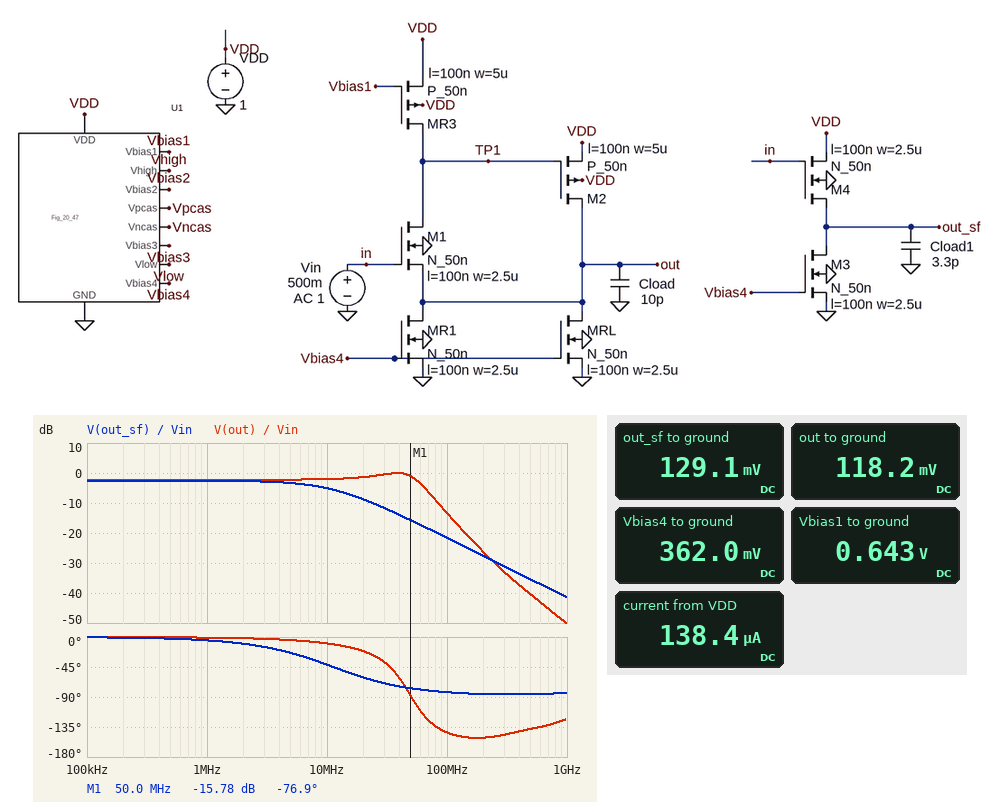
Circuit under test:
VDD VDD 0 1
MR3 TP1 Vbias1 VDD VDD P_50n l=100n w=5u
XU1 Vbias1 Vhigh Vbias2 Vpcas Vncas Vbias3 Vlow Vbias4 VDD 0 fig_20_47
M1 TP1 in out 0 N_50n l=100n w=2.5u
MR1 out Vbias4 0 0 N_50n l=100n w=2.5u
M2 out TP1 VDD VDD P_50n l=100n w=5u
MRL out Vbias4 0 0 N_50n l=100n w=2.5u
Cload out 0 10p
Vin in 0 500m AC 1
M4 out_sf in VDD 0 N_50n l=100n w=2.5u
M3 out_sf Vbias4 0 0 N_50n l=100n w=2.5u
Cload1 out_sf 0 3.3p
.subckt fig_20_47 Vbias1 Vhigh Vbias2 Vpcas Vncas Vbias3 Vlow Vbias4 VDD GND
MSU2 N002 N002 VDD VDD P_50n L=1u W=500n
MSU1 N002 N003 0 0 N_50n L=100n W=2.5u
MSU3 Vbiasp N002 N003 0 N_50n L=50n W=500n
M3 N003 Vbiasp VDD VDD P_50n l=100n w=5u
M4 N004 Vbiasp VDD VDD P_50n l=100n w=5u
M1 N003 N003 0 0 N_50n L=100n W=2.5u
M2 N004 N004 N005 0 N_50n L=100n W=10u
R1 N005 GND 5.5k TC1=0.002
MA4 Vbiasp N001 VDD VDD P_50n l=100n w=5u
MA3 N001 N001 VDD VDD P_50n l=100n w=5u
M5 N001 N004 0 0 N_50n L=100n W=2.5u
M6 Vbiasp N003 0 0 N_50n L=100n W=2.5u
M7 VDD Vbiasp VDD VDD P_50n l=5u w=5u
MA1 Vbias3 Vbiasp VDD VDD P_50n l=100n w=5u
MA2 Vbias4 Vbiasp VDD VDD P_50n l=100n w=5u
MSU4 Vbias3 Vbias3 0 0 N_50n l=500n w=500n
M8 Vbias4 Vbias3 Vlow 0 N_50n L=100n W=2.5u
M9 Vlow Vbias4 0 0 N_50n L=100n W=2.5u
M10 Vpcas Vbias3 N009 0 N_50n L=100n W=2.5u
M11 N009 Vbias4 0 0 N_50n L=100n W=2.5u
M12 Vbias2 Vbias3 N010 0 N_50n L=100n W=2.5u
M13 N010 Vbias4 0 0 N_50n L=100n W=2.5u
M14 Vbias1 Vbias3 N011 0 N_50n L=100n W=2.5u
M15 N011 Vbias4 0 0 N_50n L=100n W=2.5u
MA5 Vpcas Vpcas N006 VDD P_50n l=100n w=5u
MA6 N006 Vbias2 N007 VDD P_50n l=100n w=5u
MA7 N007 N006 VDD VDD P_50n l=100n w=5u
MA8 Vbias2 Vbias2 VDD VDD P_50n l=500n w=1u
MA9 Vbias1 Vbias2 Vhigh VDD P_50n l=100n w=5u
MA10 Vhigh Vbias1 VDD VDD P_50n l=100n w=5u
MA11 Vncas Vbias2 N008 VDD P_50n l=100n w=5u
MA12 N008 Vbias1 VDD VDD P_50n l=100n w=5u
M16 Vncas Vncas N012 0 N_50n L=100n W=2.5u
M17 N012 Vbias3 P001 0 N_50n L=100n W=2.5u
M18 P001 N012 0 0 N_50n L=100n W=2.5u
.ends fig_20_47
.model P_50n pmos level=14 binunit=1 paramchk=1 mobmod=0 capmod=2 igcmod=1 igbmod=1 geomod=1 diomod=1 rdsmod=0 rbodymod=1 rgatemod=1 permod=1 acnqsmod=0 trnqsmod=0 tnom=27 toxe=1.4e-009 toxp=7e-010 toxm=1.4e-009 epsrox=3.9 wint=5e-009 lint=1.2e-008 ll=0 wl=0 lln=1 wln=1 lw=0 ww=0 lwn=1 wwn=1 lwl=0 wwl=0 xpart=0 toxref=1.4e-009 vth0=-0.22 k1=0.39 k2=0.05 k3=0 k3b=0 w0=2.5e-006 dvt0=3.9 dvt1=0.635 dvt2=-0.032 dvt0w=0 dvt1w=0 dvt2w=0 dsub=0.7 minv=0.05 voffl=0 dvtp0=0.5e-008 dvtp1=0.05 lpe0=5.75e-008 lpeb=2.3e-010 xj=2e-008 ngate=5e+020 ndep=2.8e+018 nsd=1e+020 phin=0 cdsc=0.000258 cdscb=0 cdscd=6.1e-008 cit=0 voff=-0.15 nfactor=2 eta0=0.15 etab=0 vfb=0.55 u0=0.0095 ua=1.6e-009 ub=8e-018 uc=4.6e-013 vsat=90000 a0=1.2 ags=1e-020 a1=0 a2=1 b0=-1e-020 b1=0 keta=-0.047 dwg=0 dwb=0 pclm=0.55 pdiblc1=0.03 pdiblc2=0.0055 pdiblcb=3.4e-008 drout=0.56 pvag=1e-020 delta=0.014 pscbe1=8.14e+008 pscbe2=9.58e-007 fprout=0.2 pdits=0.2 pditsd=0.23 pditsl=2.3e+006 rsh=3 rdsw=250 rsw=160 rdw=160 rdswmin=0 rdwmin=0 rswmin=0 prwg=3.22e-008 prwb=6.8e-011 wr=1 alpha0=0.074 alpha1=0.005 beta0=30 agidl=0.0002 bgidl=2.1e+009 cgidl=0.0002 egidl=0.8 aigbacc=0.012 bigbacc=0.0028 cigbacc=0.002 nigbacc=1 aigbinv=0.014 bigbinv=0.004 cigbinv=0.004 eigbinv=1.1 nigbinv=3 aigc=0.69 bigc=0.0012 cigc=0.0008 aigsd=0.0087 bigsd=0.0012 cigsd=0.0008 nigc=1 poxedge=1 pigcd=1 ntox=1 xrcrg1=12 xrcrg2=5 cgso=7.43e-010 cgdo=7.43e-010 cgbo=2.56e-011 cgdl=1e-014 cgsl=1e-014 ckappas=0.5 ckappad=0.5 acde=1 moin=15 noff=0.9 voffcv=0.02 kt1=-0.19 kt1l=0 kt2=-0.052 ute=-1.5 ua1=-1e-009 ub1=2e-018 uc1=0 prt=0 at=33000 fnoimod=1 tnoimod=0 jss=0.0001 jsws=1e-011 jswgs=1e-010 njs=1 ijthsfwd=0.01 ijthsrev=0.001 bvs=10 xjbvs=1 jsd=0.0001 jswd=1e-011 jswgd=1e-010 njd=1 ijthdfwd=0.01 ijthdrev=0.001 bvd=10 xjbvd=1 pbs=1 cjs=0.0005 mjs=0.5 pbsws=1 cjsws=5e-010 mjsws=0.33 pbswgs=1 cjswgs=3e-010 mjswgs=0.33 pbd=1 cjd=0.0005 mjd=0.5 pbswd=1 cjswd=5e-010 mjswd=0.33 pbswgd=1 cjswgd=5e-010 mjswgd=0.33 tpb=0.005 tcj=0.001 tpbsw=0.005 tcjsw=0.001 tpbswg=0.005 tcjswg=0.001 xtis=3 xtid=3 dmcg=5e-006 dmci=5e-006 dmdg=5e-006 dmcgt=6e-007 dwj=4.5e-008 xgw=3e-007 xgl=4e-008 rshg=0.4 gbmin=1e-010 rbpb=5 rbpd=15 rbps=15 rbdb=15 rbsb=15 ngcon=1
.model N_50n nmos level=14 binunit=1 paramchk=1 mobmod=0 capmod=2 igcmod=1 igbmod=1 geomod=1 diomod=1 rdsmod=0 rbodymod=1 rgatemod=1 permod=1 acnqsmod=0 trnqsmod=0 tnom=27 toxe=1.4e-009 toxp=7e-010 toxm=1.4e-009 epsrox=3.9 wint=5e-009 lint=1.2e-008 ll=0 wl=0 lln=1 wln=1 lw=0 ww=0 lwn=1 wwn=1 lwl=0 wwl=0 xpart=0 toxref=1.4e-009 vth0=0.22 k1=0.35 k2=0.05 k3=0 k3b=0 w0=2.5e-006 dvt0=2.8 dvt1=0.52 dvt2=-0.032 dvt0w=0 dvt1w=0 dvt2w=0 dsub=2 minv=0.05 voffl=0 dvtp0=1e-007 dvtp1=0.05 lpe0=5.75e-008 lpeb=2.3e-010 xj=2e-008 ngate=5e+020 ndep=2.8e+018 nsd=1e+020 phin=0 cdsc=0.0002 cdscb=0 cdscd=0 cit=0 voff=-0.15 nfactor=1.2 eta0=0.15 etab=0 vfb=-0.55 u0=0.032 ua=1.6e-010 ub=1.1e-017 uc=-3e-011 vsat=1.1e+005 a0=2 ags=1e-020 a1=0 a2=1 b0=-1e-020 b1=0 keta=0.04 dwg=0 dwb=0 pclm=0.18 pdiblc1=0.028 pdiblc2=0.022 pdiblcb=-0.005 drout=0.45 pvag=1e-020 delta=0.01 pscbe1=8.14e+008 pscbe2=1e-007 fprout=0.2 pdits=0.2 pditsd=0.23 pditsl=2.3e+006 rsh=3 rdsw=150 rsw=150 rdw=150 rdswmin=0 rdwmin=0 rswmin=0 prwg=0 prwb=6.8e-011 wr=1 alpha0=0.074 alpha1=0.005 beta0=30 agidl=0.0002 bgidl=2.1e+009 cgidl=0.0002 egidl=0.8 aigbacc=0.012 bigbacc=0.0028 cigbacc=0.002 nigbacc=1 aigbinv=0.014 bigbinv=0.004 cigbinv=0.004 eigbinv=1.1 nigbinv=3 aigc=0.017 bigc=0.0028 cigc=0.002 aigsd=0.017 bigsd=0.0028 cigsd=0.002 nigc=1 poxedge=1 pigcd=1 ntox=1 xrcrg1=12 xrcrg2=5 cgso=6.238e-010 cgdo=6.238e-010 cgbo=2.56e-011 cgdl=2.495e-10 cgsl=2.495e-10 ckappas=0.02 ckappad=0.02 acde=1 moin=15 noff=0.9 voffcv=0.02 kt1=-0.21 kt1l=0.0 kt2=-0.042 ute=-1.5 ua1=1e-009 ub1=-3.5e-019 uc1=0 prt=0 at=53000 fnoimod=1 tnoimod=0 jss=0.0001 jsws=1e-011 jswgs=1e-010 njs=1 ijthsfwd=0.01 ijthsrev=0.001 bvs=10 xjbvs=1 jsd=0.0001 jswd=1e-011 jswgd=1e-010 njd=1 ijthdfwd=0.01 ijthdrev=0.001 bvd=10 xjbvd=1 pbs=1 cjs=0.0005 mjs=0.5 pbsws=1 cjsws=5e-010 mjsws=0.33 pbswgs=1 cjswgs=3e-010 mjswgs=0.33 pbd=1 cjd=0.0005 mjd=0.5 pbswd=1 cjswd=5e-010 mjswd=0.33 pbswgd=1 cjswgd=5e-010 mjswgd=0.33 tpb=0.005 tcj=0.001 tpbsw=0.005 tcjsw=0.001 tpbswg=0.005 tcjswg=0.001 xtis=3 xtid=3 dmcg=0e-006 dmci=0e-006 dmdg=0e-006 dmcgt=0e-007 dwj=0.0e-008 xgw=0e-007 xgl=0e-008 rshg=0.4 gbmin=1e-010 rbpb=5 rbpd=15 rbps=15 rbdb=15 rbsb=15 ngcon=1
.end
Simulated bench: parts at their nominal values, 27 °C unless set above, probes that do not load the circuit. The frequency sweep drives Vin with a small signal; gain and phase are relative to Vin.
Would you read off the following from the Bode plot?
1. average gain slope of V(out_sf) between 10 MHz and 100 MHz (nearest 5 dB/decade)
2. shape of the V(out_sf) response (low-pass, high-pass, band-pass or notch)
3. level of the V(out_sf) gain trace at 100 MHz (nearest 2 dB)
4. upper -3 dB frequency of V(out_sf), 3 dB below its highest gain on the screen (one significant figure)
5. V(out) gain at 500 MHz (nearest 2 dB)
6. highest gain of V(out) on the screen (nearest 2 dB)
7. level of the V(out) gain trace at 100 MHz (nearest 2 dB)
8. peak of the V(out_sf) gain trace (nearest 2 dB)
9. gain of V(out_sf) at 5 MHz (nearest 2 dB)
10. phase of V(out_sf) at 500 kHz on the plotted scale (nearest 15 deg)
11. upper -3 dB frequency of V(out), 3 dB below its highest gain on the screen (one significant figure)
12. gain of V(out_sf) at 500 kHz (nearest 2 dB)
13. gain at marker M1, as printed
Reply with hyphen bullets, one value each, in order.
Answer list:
- -15 dB/decade
- low-pass
- -22 dB
- 10 MHz
- -40 dB
- 0 dB
- -14 dB
- -2 dB
- -4 dB
- 0 deg
- 60 MHz
- -2 dB
- -15.78 dB
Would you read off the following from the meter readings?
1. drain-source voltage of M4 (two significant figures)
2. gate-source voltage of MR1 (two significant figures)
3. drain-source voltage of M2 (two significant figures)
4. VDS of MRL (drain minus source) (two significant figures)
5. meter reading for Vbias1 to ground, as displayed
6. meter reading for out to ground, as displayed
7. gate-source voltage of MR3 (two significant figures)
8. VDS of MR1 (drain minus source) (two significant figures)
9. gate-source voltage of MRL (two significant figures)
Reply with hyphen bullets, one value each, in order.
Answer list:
- -870 mV
- 360 mV
- -880 mV
- 120 mV
- 0.643 V
- 118.2 mV
- -360 mV
- 120 mV
- 360 mV
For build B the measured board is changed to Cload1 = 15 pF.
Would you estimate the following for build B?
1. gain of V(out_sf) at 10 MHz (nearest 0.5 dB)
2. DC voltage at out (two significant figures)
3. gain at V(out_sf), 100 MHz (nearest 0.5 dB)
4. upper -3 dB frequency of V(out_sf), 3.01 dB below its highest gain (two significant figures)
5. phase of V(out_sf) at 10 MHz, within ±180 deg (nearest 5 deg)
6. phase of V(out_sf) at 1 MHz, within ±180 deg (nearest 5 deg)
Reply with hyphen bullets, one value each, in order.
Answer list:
- -15.0 dB
- 120 mV
- -34.5 dB
- 2.5 MHz
- -75 deg
- -20 deg
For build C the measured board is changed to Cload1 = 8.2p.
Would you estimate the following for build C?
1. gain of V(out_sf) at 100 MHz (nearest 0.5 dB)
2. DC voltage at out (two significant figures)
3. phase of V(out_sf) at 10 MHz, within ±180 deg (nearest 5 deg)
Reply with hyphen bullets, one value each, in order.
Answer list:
- -29.5 dB
- 120 mV
- -65 deg
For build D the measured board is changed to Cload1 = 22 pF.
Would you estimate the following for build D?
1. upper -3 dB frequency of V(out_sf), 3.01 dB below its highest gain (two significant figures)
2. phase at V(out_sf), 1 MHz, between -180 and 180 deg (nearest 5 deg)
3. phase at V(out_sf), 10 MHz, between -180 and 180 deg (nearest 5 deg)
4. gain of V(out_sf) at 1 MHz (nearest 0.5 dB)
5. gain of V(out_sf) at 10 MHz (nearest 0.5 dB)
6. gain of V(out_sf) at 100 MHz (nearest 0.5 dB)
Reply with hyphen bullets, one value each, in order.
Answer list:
- 1.7 MHz
- -30 deg
- -80 deg
- -4.0 dB
- -18.0 dB
- -38.0 dB
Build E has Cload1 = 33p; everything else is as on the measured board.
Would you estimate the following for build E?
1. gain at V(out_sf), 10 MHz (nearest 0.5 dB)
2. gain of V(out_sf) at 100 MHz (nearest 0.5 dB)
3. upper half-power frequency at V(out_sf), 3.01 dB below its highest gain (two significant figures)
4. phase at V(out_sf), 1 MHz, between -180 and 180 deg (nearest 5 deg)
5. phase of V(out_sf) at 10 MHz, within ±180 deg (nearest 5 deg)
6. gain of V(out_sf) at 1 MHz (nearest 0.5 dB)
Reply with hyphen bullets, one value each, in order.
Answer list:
- -21.5 dB
- -41.5 dB
- 1.1 MHz
- -40 deg
- -85 deg
- -5.0 dB
